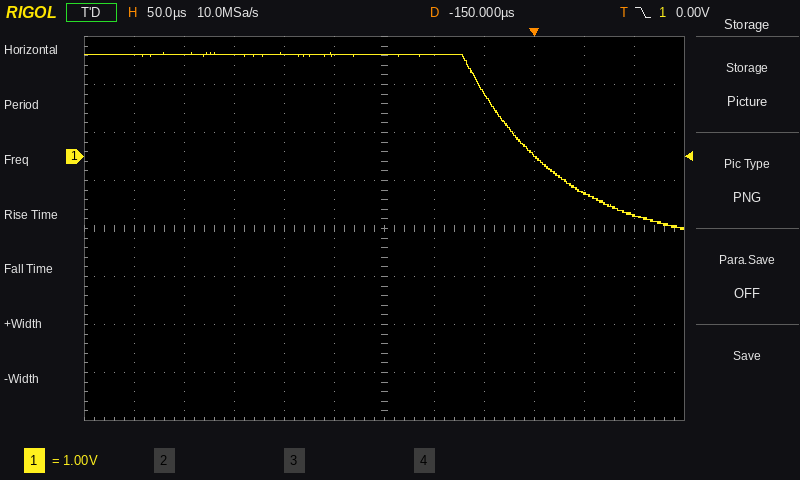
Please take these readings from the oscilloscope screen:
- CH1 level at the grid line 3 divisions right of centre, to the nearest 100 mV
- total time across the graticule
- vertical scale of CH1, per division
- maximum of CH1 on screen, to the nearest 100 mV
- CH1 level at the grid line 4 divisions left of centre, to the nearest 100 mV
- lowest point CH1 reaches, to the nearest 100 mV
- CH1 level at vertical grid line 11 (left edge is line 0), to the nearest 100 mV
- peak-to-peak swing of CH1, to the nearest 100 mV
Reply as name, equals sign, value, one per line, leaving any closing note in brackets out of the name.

CH1 level at the grid line 3 divisions right of centre, to the nearest 100 mV = 0.0 V
total time across the graticule = 600 µs
vertical scale of CH1, per division = 1 V
maximum of CH1 on screen, to the nearest 100 mV = 2.2 V
CH1 level at the grid line 4 divisions left of centre, to the nearest 100 mV = 2.1 V
lowest point CH1 reaches, to the nearest 100 mV = -1.5 V
CH1 level at vertical grid line 11 (left edge is line 0), to the nearest 100 mV = -1.2 V
peak-to-peak swing of CH1, to the nearest 100 mV = 3.7 V
